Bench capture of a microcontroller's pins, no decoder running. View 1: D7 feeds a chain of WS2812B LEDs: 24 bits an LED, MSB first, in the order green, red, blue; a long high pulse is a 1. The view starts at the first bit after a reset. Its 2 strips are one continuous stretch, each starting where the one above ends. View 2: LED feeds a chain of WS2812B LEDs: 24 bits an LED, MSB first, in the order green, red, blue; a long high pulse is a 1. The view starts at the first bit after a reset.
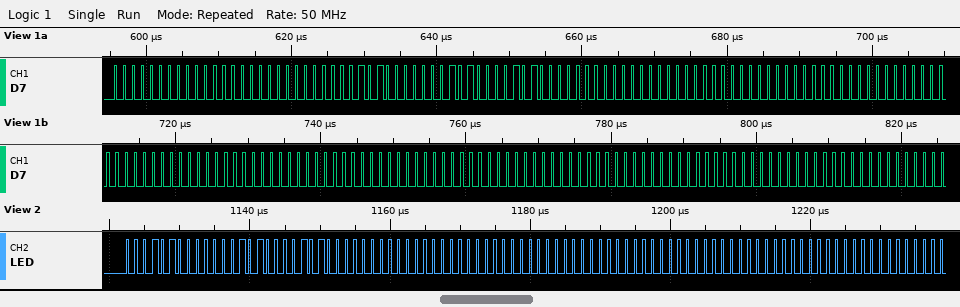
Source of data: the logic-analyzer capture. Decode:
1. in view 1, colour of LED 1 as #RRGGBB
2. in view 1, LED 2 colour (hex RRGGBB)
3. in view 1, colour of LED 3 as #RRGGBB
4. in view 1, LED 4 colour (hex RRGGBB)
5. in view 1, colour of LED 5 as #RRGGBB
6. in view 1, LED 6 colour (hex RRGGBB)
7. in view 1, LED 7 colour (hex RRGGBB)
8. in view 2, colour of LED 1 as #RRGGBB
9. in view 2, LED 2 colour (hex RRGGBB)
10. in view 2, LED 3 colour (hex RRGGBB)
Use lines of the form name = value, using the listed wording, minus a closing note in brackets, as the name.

in view 1, colour of LED 1 as #RRGGBB = #000000
in view 1, LED 2 colour = #05140A
in view 1, colour of LED 3 as #RRGGBB = #000000
in view 1, LED 4 colour = #000000
in view 1, colour of LED 5 as #RRGGBB = #000000
in view 1, LED 6 colour = #000000
in view 1, LED 7 colour = #000000
in view 2, colour of LED 1 as #RRGGBB = #05140A
in view 2, LED 2 colour = #000000
in view 2, LED 3 colour = #000000
